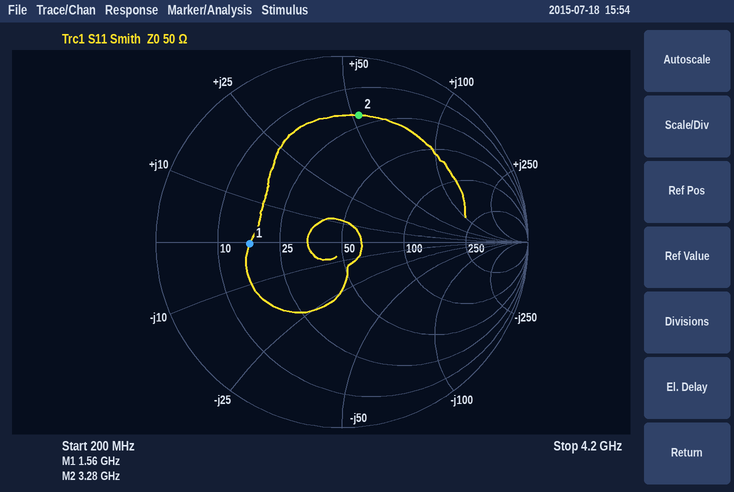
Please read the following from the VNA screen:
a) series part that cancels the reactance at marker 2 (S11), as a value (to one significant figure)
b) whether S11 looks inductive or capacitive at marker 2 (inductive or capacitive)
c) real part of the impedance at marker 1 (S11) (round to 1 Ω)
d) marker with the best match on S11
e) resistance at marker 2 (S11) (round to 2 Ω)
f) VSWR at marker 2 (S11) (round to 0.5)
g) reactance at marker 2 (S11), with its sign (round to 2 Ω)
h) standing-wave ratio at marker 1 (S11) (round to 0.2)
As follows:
900 fF
inductive
17 Ω
marker 1
20 Ω
5.5
+52 Ω
3.0
